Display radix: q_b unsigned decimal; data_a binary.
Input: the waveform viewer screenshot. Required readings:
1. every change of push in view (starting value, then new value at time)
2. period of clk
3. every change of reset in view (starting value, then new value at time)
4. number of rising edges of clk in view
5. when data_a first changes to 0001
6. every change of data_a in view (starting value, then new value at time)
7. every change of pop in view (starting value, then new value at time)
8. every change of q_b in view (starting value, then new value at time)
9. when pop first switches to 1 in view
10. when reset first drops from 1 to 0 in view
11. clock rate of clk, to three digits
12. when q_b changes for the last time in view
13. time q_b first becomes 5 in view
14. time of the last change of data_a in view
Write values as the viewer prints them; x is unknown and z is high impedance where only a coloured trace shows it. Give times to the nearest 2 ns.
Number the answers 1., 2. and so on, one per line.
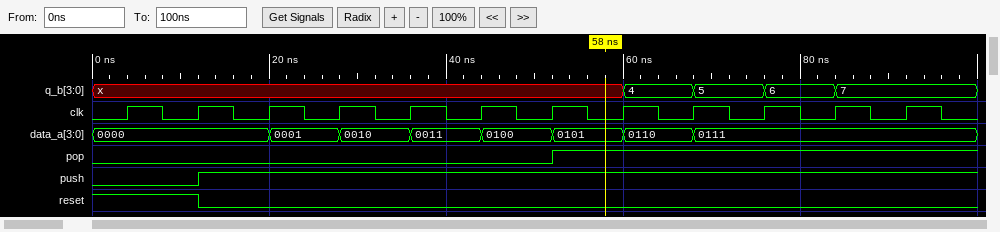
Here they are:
1. 0, 1 at 12 ns
2. 8 ns
3. 1, 0 at 12 ns
4. 12
5. 20 ns
6. 0000, 0001 at 20 ns, 0010 at 28 ns, 0011 at 36 ns, 0100 at 44 ns, 0101 at 52 ns, 0110 at 60 ns, 0111 at 68 ns
7. 0, 1 at 52 ns
8. x, 4 at 60 ns, 5 at 68 ns, 6 at 76 ns, 7 at 84 ns
9. 52 ns
10. 12 ns
11. 125 MHz
12. 84 ns
13. 68 ns
14. 68 ns
